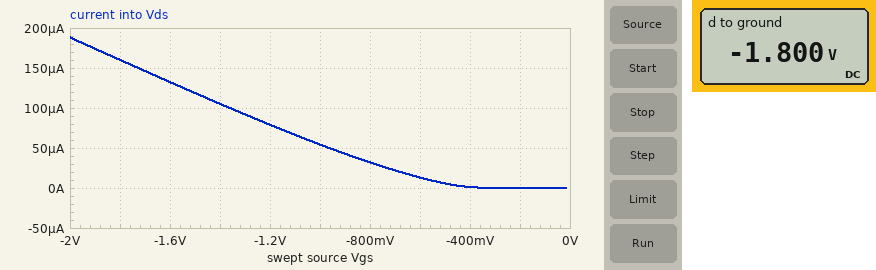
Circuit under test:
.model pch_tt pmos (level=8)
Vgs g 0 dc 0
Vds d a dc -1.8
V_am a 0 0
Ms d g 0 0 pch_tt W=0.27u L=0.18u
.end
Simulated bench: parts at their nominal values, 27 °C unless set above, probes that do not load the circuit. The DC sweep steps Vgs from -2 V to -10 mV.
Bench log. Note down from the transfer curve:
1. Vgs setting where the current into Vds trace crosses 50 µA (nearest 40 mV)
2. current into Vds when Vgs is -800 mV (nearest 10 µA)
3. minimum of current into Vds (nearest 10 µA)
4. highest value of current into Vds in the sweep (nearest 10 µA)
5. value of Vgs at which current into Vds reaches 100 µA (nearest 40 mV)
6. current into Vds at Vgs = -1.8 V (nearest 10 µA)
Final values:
-960 mV
30 µA
0 A
190 µA
-1.36 V
160 µA
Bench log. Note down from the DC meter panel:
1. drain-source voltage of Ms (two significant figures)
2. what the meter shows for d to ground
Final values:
-1.8 V
-1.800 V
